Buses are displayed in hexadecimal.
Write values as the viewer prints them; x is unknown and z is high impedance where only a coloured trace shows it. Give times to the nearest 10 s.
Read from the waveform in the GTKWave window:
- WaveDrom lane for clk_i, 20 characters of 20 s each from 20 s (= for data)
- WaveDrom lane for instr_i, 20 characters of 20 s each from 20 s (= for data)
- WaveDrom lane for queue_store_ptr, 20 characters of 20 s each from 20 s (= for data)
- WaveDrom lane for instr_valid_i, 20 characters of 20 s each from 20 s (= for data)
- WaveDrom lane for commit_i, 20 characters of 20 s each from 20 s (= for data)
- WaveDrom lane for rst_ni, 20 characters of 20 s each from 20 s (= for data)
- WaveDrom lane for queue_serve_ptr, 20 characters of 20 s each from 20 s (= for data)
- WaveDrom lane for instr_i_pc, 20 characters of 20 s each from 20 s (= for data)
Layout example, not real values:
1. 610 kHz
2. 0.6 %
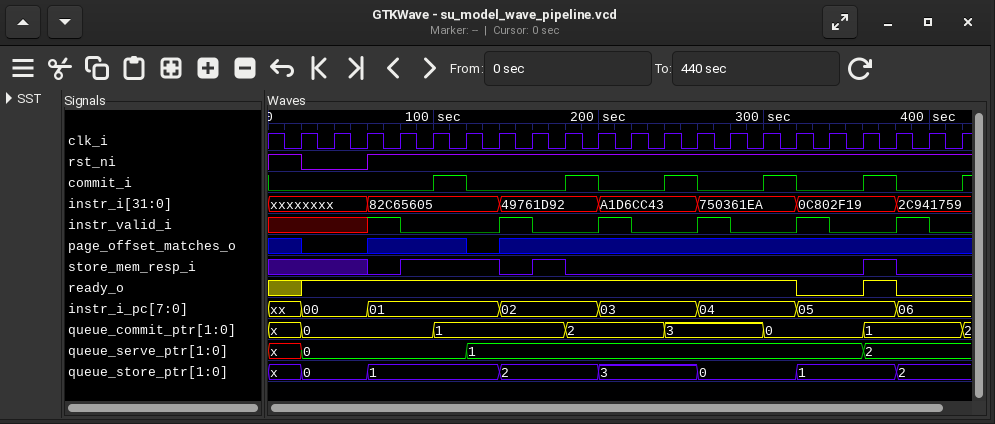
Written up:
1. {name: 'clk_i', wave: 'p...................'}
2. {name: 'instr_i', wave: 'x.=...=..=..=..=..=.', data: '82C65605 49761D92 A1D6CC43 750361EA 0C802F19 2C941759'}
3. {name: 'queue_store_ptr', wave: '=.=...=..=..=..=..=.', data: '0 1 2 3 0 1 2'}
4. {name: 'instr_valid_i', wave: 'x.10..10.10.10.10.10'}
5. {name: 'commit_i', wave: '0...10..10.10.10.10.'}
6. {name: 'rst_ni', wave: '0.1.................'}
7. {name: 'queue_serve_ptr', wave: '=....=...........=..', data: '0 1 2'}
8. {name: 'instr_i_pc', wave: '=.=...=..=..=..=..=.', data: '00 01 02 03 04 05 06'}
